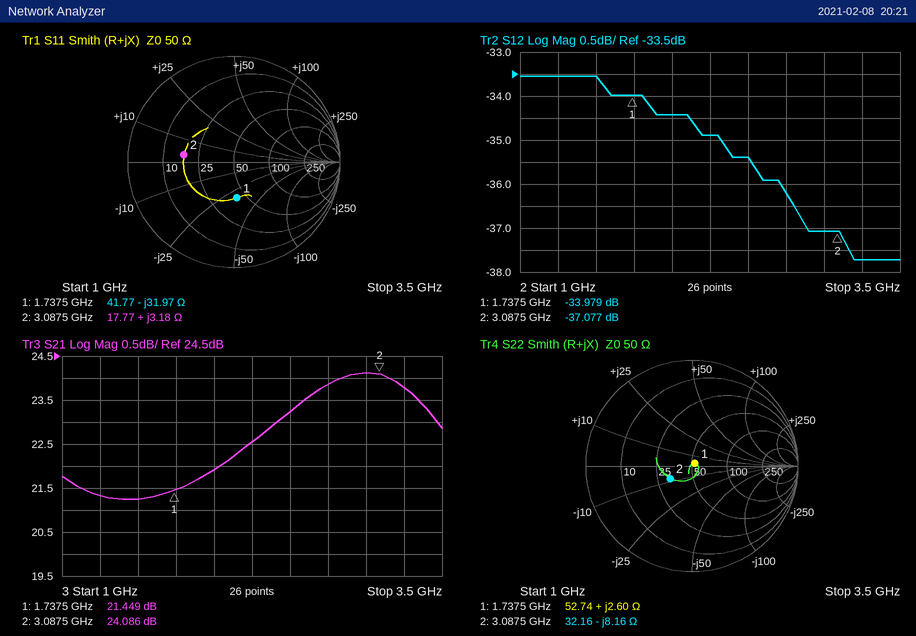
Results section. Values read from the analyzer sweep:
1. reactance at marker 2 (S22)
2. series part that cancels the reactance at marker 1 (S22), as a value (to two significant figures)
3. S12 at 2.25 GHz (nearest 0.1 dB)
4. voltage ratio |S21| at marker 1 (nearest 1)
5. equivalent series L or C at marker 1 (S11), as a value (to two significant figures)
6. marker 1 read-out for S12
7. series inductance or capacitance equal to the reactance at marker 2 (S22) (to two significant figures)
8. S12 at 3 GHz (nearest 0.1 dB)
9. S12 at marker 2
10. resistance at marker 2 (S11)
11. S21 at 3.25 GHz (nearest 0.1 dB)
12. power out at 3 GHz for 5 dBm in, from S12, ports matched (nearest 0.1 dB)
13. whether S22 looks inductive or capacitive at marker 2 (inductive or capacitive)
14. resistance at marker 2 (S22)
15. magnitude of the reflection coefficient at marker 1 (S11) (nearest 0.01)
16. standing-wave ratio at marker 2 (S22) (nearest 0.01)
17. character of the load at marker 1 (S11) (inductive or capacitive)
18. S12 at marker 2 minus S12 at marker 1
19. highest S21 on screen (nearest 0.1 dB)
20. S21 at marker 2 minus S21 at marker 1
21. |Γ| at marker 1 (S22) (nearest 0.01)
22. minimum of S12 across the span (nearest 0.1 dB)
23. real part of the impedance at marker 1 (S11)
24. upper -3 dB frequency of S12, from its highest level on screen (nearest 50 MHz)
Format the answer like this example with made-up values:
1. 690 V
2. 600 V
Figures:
1. -8.16 Ω
2. 35 pF
3. -34.9 dB
4. 12
5. 2.9 pF
6. -33.979 dB
7. 6.3 pF
8. -37.1 dB
9. -37.077 dB
10. 17.77 Ω
11. 23.8 dB
12. -32.1 dBm
13. capacitive
14. 32.16 Ω
15. 0.34
16. 1.62
17. capacitive
18. -3.098 dB
19. 24.1 dB
20. 2.637 dB
21. 0.04
22. -37.7 dB
23. 41.77 Ω
24. 2.80 GHz
